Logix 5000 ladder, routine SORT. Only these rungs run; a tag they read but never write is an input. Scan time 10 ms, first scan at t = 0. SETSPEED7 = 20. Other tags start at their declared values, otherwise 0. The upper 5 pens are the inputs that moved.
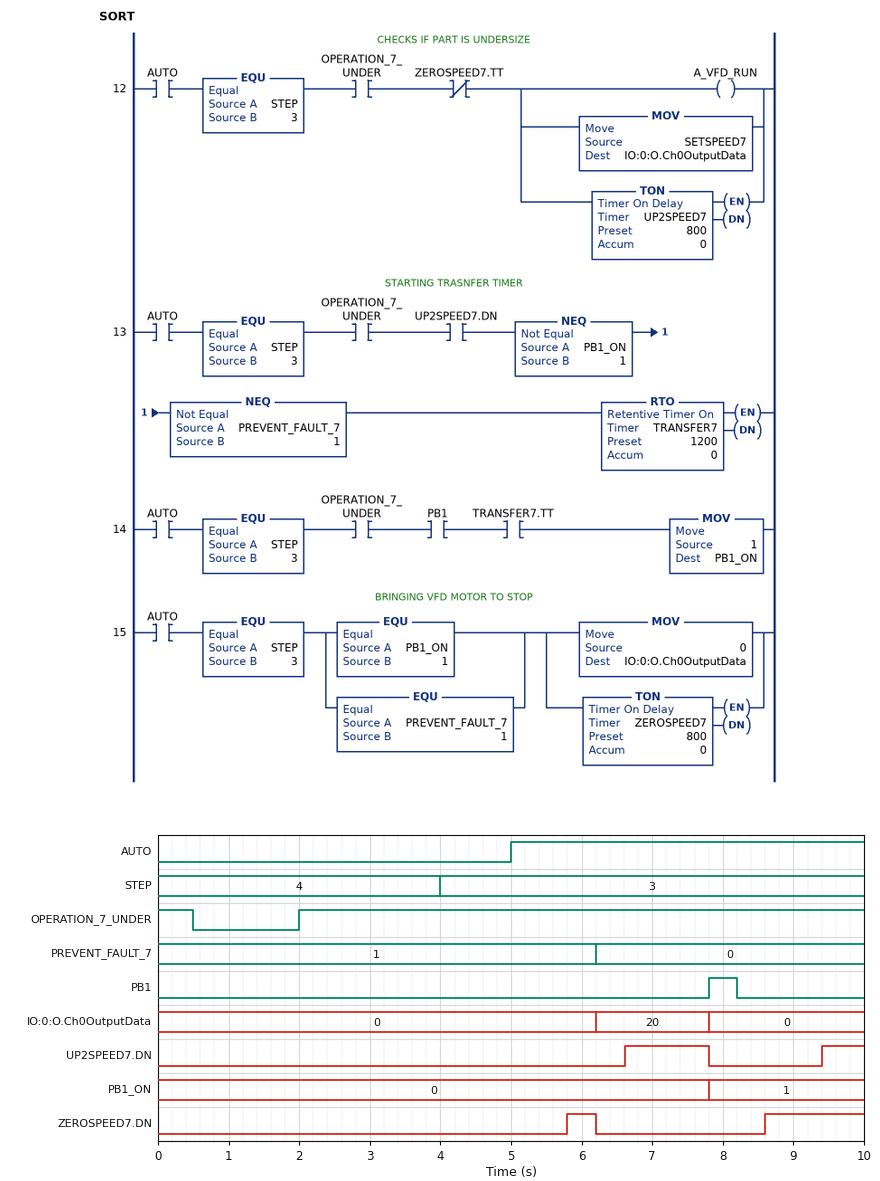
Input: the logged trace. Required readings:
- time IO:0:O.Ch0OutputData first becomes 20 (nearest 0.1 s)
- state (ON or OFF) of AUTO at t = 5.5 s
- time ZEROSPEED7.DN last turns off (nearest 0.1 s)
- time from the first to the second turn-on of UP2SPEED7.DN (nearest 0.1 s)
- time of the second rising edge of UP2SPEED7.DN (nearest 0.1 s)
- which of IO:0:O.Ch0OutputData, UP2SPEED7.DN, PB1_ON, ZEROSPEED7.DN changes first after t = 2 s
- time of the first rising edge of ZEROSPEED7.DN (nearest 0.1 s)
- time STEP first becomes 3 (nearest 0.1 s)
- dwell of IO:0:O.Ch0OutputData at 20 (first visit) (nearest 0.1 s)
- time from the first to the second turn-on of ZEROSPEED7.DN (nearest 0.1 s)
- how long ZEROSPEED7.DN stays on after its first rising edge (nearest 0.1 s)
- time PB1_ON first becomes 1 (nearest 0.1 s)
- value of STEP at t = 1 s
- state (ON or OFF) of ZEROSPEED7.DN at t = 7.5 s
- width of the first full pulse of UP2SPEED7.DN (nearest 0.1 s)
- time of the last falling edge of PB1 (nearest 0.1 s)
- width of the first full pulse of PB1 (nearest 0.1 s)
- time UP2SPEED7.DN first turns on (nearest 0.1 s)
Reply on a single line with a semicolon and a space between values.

6.2 s; ON; 6.2 s; 2.8 s; 9.4 s; ZEROSPEED7.DN; 5.8 s; 4.0 s; 1.6 s; 2.8 s; 0.4 s; 7.8 s; 4; OFF; 1.2 s; 8.2 s; 0.4 s; 6.6 s
